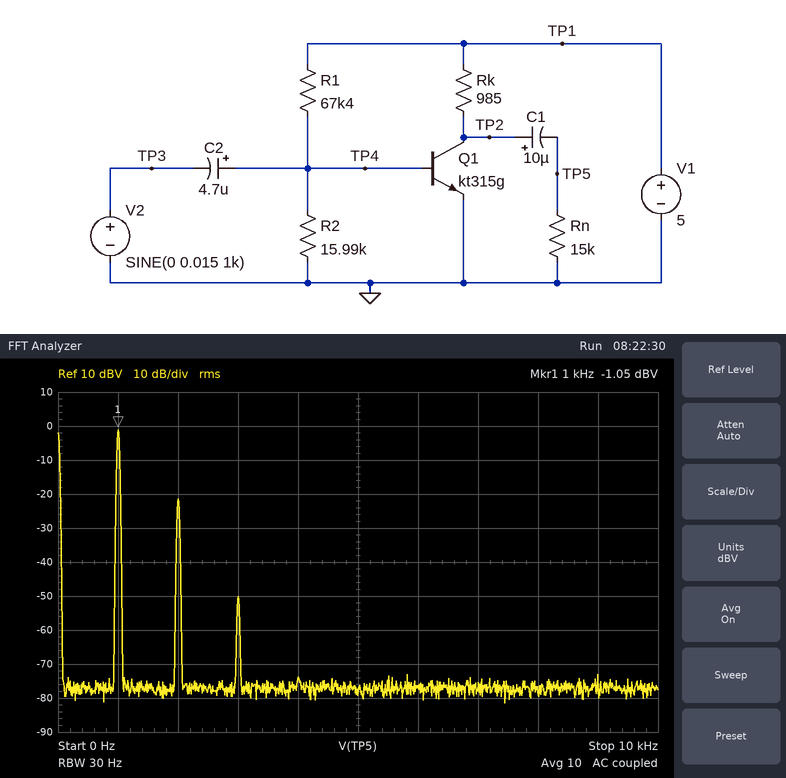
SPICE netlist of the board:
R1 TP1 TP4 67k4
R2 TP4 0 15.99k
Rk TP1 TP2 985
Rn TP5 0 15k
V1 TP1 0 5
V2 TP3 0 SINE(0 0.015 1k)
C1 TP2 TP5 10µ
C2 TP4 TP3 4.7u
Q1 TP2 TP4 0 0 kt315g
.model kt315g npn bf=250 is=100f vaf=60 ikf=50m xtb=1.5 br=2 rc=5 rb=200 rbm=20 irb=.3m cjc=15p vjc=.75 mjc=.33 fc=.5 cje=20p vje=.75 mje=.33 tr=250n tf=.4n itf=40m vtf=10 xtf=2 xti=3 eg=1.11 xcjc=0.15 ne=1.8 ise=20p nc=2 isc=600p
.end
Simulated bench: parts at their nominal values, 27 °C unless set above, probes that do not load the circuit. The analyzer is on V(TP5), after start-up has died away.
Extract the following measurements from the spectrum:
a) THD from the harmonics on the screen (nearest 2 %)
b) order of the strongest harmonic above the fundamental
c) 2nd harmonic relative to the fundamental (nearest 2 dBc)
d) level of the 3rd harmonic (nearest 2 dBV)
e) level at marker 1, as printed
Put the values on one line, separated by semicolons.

10 %; 2; -20 dBc; -50 dBV; -1.05 dBV
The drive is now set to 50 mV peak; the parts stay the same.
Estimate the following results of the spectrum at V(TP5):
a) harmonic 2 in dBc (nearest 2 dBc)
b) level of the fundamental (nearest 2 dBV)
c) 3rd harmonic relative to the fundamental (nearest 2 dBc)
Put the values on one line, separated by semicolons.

-12 dBc; 4 dBV; -32 dBc
